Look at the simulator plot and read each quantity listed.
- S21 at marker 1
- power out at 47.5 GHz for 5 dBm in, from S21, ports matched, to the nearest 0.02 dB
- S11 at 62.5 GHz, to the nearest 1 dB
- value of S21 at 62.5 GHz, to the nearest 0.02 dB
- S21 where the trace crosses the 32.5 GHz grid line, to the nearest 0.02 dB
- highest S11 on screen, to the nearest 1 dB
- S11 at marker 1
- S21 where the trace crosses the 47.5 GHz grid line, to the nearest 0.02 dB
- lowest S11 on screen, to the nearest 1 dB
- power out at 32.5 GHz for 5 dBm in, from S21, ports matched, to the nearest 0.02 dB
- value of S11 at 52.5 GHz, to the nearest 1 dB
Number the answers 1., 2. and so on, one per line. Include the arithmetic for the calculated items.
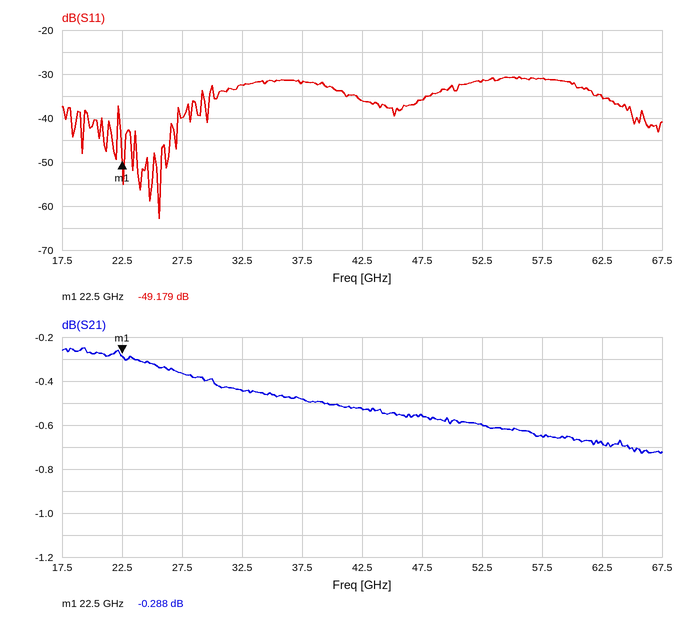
1. -0.288 dB
2. 5 dBm + (-0.56 dB) = 4.44 dBm
3. -35 dB
4. -0.68 dB
5. -0.44 dB
6. -31 dB
7. -49.179 dB
8. -0.56 dB
9. -63 dB
10. 5 dBm + (-0.44 dB) = 4.56 dBm
11. -32 dB
